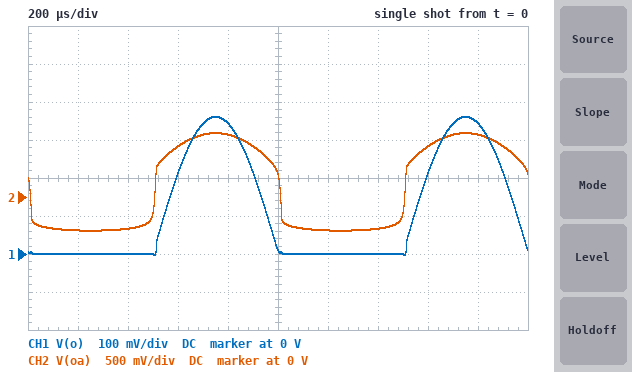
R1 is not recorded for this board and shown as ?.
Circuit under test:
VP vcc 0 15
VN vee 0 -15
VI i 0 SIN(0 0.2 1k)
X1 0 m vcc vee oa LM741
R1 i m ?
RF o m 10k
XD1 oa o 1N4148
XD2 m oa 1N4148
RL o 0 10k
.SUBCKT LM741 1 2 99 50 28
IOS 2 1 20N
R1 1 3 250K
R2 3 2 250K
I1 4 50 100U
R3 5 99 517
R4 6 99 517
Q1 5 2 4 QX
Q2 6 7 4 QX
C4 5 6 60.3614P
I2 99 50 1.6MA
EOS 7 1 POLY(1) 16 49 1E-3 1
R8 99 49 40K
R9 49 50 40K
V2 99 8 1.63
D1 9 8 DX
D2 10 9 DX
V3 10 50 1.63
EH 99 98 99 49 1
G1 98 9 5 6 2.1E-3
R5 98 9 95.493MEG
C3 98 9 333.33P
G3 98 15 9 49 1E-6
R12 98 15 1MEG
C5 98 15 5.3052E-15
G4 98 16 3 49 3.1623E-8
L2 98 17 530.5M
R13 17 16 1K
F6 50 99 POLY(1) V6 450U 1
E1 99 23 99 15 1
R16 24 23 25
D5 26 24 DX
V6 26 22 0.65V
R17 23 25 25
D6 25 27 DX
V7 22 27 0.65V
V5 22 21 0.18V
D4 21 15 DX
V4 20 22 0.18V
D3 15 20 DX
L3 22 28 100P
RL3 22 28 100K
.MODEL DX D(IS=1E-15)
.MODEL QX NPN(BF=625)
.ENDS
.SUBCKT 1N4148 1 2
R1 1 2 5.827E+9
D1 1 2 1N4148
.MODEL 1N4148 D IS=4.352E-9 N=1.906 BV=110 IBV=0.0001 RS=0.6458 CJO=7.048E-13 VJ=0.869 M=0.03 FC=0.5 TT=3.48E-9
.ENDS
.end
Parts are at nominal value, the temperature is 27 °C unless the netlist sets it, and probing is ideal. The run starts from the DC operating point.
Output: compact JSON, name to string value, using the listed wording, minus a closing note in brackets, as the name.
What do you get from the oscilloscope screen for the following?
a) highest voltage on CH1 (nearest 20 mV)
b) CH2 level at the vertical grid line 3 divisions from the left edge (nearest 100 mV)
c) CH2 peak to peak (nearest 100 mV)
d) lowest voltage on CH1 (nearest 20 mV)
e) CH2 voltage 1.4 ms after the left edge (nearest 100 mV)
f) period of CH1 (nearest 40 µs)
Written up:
{"highest voltage on CH1": "360 mV", "CH2 level at the vertical grid line 3 divisions from the left edge": "700 mV", "CH2 peak to peak": "1.3 V", "lowest voltage on CH1": "0 V", "CH2 voltage 1.4 ms after the left edge": "-400 mV", "period of CH1": "1.00 ms"}
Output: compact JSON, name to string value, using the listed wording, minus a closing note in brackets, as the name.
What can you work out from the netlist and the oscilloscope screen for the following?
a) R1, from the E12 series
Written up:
{"R1, from the E12 series": "5.6 kΩ"}
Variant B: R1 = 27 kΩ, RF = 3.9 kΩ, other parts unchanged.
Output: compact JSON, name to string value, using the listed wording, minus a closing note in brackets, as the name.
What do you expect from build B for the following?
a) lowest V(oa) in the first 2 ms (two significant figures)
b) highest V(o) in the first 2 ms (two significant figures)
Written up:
{"lowest V(oa) in the first 2 ms": "-360 mV", "highest V(o) in the first 2 ms": "30 mV"}
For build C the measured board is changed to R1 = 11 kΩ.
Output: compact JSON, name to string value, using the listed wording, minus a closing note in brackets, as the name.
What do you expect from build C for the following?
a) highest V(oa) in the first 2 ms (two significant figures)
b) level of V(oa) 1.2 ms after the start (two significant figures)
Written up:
{"highest V(oa) in the first 2 ms": "630 mV", "level of V(oa) 1.2 ms after the start": "-410 mV"}
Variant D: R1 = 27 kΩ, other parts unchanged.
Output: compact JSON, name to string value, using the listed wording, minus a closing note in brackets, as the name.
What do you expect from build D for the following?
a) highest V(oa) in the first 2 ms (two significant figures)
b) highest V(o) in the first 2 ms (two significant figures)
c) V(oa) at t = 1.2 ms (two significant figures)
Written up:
{"highest V(oa) in the first 2 ms": "480 mV", "highest V(o) in the first 2 ms": "76 mV", "V(oa) at t = 1.2 ms": "-360 mV"}
